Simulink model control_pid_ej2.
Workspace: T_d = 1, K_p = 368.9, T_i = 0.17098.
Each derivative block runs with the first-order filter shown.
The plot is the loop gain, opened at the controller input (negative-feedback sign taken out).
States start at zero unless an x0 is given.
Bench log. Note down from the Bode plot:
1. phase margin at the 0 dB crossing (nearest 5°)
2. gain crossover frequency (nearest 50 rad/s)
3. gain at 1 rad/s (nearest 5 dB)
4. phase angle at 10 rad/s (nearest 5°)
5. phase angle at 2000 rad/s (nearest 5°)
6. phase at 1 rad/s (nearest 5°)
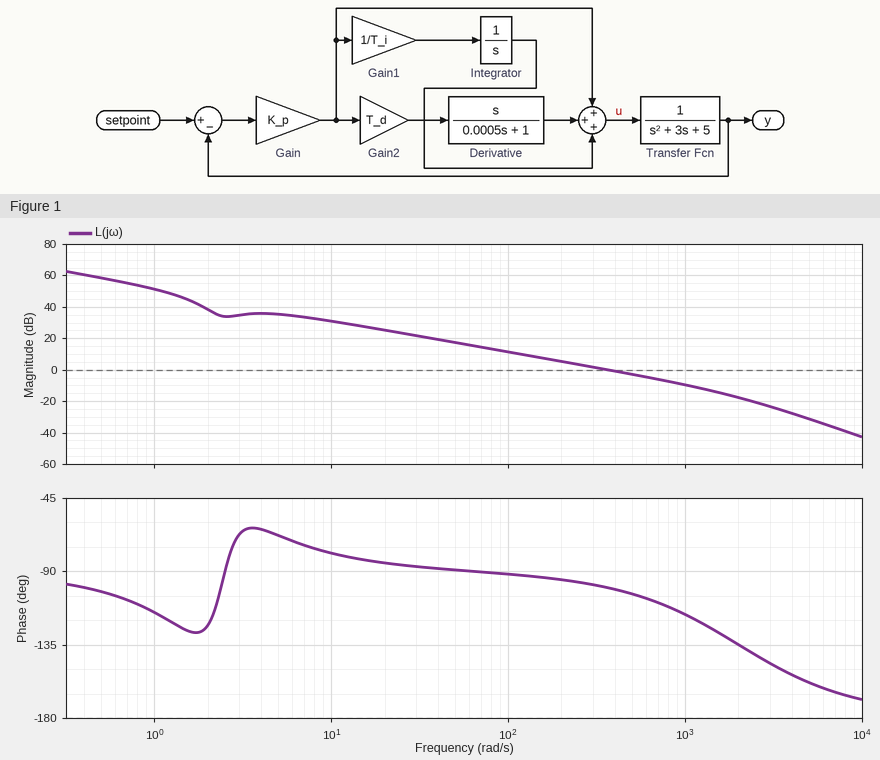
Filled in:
80°
350 rad/s
50 dB
-80°
-135°
-115°
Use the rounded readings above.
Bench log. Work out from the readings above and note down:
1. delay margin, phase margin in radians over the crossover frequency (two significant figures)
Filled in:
0.0040 s
